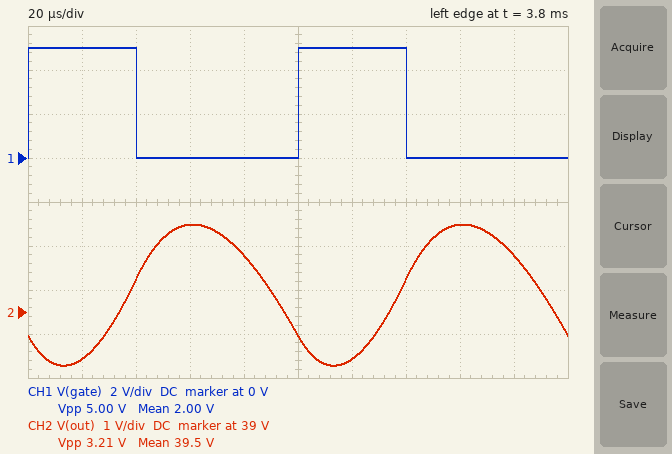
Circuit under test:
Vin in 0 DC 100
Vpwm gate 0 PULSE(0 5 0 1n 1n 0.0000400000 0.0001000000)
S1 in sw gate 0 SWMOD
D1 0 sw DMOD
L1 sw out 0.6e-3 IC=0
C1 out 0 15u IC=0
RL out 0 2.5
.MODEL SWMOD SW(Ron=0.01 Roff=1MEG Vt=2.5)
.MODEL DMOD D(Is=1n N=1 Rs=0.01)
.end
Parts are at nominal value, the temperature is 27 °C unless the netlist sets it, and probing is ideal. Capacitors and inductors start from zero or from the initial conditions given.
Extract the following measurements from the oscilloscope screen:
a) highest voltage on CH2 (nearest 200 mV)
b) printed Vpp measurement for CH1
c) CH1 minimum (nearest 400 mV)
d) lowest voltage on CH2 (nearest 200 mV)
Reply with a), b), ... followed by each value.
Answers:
a) 41.0 V
b) 5.00 V
c) 0 V
d) 37.8 V
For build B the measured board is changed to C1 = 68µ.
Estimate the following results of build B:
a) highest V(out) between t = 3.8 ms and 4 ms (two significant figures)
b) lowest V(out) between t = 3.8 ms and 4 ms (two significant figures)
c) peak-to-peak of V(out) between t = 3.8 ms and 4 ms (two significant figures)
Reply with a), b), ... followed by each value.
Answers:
a) 40 V
b) 39 V
c) 740 mV
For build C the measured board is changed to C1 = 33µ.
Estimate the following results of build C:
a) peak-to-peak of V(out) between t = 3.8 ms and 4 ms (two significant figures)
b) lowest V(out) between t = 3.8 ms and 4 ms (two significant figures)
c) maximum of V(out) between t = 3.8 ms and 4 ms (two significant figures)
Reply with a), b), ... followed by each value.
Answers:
a) 1.5 V
b) 39 V
c) 40 V
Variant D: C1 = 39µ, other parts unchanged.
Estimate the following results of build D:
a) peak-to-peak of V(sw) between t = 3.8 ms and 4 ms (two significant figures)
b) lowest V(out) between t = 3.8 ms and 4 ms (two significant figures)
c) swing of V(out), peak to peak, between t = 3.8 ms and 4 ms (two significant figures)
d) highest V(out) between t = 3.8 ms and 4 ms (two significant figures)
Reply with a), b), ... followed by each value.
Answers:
a) 100 V
b) 39 V
c) 1.3 V
d) 40 V
